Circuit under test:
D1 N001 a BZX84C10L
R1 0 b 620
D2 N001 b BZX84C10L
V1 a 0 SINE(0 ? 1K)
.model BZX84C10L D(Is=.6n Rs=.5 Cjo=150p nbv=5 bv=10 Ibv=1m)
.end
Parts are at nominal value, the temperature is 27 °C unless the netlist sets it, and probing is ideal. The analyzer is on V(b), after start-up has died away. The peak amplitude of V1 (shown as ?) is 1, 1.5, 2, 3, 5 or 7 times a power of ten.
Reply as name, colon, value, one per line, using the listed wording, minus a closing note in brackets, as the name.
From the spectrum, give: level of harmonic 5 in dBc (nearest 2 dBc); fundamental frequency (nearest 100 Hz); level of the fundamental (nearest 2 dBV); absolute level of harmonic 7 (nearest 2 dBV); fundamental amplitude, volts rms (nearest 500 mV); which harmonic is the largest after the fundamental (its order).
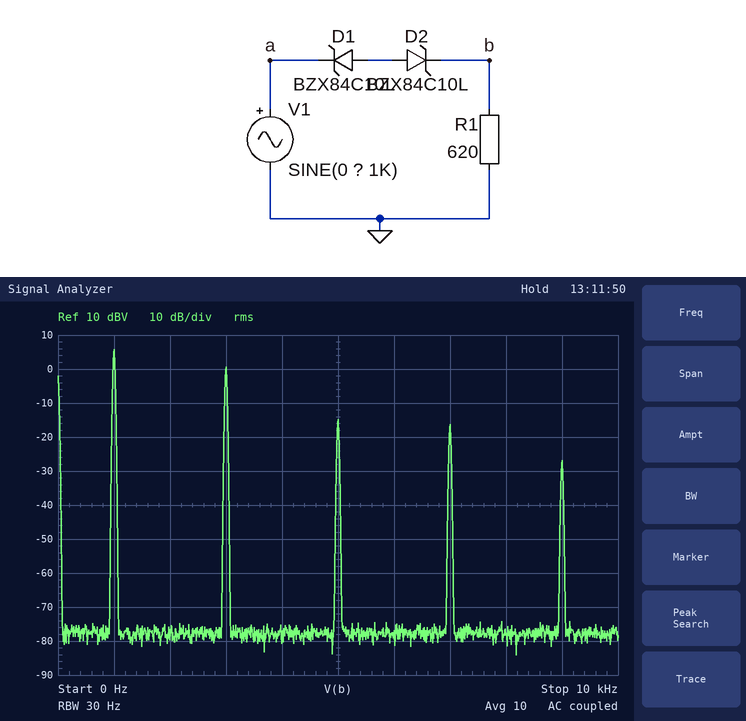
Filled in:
level of harmonic 5 in dBc: -20 dBc
fundamental frequency: 1.0 kHz
level of the fundamental: 6 dBV
absolute level of harmonic 7: -16 dBV
fundamental amplitude, volts rms: 2.0 V
which harmonic is the largest after the fundamental: 3
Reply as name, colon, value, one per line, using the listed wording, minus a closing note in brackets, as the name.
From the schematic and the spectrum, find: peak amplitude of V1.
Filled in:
peak amplitude of V1: 15 V
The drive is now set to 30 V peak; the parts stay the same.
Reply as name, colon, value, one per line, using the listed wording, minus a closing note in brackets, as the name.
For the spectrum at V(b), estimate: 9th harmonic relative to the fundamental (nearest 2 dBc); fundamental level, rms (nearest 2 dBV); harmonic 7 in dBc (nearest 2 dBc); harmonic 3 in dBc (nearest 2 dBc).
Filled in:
9th harmonic relative to the fundamental: -60 dBc
fundamental level, rms: 22 dBV
harmonic 7 in dBc: -32 dBc
harmonic 3 in dBc: -14 dBc
